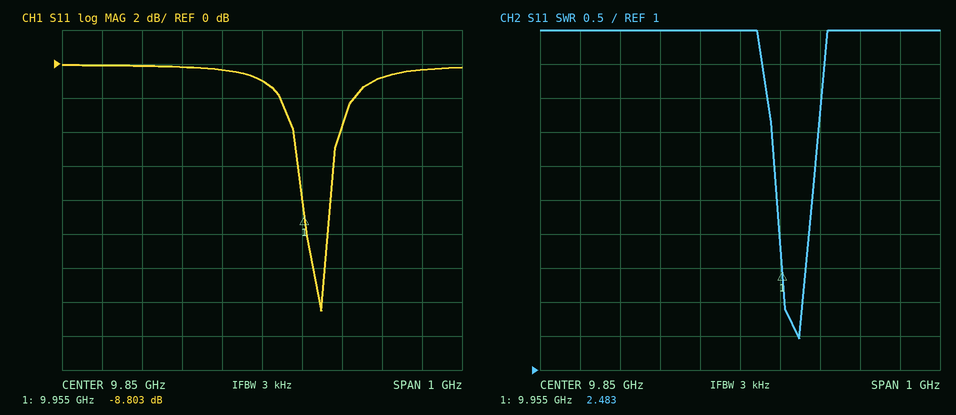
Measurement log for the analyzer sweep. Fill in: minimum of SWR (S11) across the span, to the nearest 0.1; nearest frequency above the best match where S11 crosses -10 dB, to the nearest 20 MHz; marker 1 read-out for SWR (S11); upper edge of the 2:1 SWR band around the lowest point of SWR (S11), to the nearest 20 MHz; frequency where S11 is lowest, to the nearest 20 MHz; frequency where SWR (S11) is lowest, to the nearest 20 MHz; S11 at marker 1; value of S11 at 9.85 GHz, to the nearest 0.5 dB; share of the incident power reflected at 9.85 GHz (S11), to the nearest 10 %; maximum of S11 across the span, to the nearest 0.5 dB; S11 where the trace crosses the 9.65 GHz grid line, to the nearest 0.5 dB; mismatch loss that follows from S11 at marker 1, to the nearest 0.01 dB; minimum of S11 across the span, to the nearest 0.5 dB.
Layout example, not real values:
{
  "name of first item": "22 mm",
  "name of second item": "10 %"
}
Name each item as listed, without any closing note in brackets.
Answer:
{
  "minimum of SWR (S11) across the span, to the nearest 0.1": "1.5",
  "nearest frequency above the best match where S11 crosses -10 dB, to the nearest 20 MHz": "10.02 GHz",
  "marker 1 read-out for SWR": "2.483",
  "upper edge of the 2:1 SWR band around the lowest point of SWR (S11), to the nearest 20 MHz": "10.00 GHz",
  "frequency where S11 is lowest, to the nearest 20 MHz": "10.00 GHz",
  "frequency where SWR (S11) is lowest, to the nearest 20 MHz": "10.00 GHz",
  "S11 at marker 1": "-8.803 dB",
  "value of S11 at 9.85 GHz, to the nearest 0.5 dB": "-1.0 dB",
  "share of the incident power reflected at 9.85 GHz (S11), to the nearest 10 %": "80 %",
  "maximum of S11 across the span, to the nearest 0.5 dB": "0.0 dB",
  "S11 where the trace crosses the 9.65 GHz grid line, to the nearest 0.5 dB": "0.0 dB",
  "mismatch loss that follows from S11 at marker 1, to the nearest 0.01 dB": "0.61 dB",
  "minimum of S11 across the span, to the nearest 0.5 dB": "-14.5 dB"
}
